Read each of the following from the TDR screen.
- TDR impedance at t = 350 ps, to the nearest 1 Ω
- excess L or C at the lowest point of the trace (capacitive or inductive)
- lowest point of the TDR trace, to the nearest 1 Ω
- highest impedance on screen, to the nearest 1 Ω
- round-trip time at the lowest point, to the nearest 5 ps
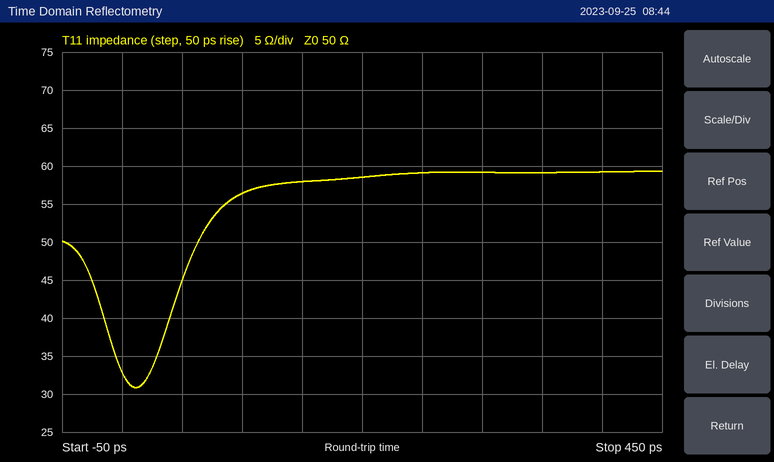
59 Ω
capacitive
31 Ω
59 Ω
10 ps
